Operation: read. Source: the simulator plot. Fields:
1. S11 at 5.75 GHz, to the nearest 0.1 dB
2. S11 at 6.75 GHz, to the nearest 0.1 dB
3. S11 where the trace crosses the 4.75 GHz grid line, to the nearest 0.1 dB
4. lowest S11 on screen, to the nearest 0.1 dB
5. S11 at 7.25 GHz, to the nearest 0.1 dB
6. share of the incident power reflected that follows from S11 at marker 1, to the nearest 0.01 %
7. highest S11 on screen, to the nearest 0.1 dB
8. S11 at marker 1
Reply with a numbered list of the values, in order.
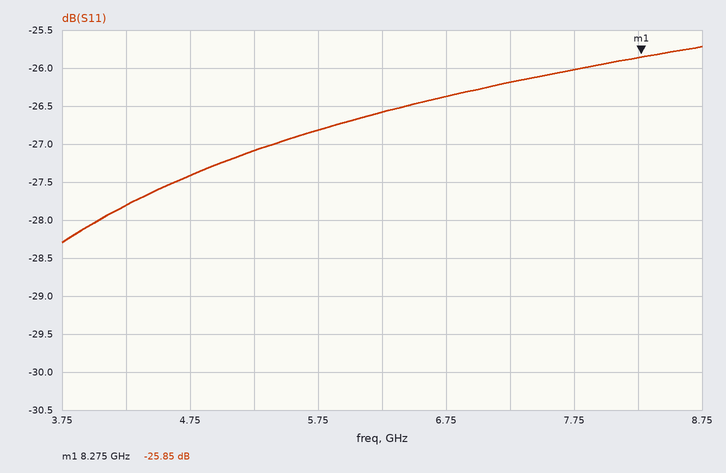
1. -26.8 dB
2. -26.4 dB
3. -27.4 dB
4. -28.3 dB
5. -26.2 dB
6. 0.26 %
7. -25.7 dB
8. -25.85 dB
